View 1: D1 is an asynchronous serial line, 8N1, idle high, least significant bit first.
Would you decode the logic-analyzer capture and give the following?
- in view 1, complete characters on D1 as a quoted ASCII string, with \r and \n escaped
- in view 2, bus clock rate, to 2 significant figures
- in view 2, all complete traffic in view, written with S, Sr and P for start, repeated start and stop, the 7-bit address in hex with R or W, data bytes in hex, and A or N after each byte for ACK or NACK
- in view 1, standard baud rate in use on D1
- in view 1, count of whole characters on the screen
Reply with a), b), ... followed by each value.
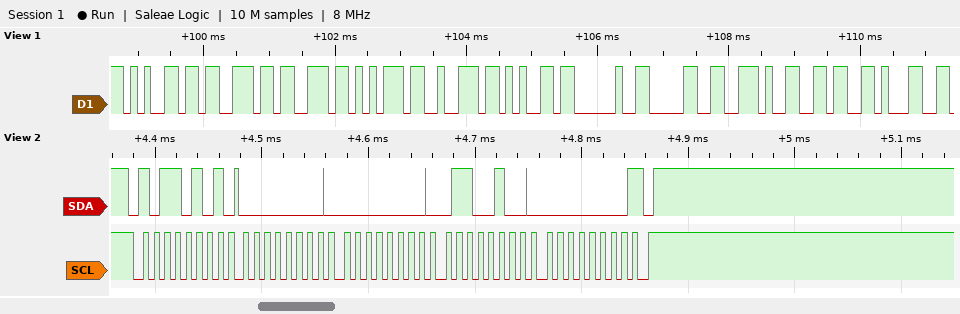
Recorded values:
a) "essure 0.61"
b) 100 kHz
c) S 5AR A 00 A 00 A 64 A 00 N P
d) 9600 baud
e) 11
